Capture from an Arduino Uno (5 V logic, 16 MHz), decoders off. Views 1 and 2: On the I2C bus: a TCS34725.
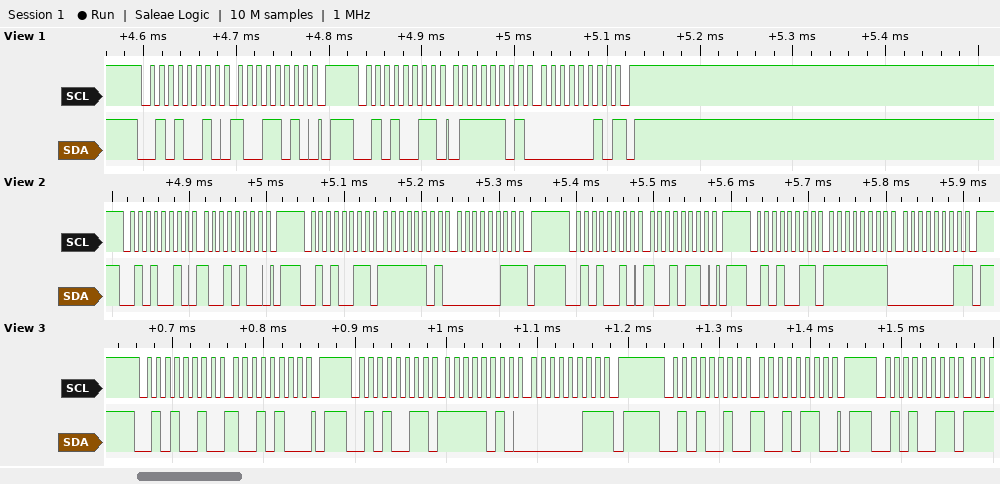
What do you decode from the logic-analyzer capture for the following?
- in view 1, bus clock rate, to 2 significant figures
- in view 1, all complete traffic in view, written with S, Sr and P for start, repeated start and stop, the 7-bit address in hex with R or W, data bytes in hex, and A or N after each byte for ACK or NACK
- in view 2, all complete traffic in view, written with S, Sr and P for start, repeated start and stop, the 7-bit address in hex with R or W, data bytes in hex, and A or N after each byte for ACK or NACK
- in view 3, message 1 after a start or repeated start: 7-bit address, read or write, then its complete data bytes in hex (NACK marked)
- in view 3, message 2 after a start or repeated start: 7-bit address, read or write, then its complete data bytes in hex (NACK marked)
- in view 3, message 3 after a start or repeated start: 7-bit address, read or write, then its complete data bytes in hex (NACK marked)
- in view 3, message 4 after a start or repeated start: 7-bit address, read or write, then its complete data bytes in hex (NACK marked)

100 kHz
S 29W A 9A A P S 29R A 7D A 02 N P
S 29W A 94 A P S 29R A FD A 03 N P S 29W A 96 A P S 29R A FF A 01 N P
0x29 write: 94
0x29 read: FA 03 NACK
0x29 write: 96
0x29 read
